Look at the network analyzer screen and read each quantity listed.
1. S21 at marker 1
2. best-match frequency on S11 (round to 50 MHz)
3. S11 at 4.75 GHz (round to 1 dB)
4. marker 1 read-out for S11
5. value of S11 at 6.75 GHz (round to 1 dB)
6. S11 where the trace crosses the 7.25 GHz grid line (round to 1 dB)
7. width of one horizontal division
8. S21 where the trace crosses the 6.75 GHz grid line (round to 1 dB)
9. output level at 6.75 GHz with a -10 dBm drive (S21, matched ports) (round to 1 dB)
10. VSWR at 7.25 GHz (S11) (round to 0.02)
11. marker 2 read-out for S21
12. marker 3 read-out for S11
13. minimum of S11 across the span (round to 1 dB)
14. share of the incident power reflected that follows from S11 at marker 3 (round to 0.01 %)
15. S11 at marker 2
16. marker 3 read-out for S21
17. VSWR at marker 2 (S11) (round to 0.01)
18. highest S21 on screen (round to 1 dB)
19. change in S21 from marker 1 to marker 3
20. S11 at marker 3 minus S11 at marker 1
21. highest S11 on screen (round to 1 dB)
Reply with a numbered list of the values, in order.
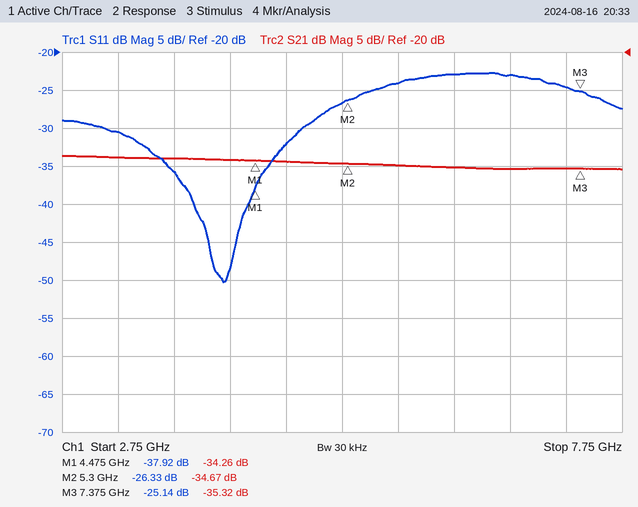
1. -34.26 dB
2. 4.20 GHz
3. -32 dB
4. -37.92 dB
5. -23 dB
6. -25 dB
7. 500 MHz
8. -35 dB
9. -45 dBm
10. 1.12
11. -34.67 dB
12. -25.14 dB
13. -50 dB
14. 0.31 %
15. -26.33 dB
16. -35.32 dB
17. 1.10
18. -34 dB
19. -1.06 dB
20. 12.78 dB
21. -23 dB
